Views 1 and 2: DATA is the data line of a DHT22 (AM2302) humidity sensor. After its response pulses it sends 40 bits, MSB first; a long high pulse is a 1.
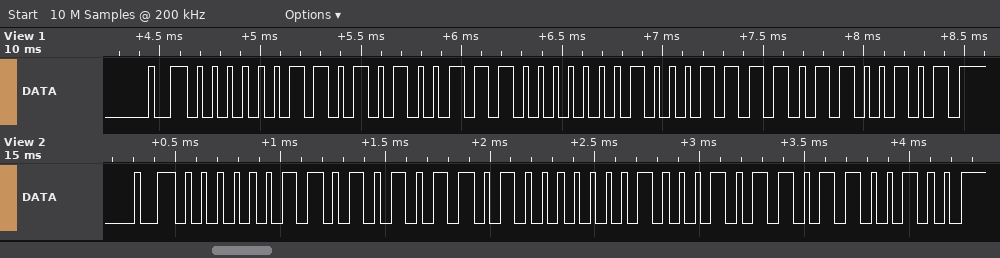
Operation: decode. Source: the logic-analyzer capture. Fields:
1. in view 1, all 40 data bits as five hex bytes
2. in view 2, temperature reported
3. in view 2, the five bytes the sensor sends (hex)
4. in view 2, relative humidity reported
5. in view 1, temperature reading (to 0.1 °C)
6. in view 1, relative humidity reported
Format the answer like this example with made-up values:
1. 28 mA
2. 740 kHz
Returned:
1. 03 53 80 8F 65
2. -13.9 °C
3. 03 56 80 8B 64
4. 85.4 %
5. -14.3 °C
6. 85.1 %
